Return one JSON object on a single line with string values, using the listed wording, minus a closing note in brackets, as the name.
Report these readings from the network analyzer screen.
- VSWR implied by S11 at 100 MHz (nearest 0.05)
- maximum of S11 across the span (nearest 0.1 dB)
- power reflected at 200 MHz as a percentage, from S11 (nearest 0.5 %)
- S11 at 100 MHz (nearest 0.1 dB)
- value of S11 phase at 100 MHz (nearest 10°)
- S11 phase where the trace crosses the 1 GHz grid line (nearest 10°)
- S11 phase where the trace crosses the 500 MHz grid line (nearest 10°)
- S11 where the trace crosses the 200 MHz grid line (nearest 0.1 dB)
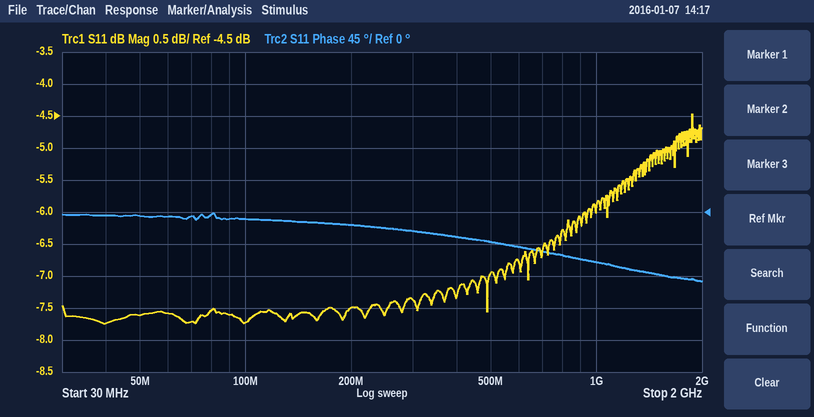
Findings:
{"VSWR implied by S11 at 100 MHz": "2.40", "maximum of S11 across the span": "-4.5 dB", "power reflected at 200 MHz as a percentage, from S11": "18.0 %", "S11 at 100 MHz": "-7.7 dB", "value of S11 phase at 100 MHz": "-10°", "S11 phase where the trace crosses the 1 GHz grid line": "-70°", "S11 phase where the trace crosses the 500 MHz grid line": "-40°", "S11 where the trace crosses the 200 MHz grid line": "-7.5 dB"}
